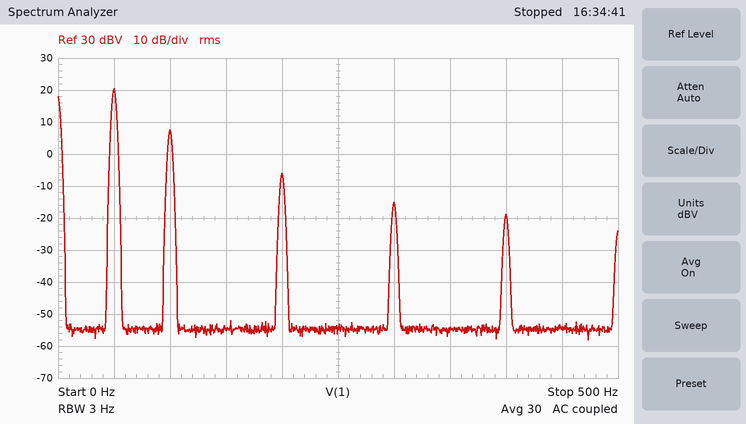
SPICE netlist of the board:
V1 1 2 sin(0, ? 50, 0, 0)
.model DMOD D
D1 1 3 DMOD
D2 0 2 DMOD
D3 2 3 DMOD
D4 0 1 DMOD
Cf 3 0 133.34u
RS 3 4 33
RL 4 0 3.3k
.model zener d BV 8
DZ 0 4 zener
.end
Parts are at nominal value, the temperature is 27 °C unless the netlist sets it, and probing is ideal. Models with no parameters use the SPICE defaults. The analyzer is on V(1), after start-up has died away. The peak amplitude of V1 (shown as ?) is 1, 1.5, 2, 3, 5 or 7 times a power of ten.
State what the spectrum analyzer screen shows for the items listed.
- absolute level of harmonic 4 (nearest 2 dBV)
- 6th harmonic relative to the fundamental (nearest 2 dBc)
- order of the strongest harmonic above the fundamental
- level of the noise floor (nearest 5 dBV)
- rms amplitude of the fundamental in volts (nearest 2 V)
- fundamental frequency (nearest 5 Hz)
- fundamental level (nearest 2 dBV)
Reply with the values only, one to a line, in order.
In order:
-6 dBV
-36 dBc
2
-55 dBV
10 V
50 Hz
20 dBV
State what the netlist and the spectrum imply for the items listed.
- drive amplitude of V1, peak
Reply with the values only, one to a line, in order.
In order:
30 V
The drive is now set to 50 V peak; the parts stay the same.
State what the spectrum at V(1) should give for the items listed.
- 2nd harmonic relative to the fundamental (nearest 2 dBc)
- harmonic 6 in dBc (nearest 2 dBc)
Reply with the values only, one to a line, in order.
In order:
-12 dBc
-34 dBc
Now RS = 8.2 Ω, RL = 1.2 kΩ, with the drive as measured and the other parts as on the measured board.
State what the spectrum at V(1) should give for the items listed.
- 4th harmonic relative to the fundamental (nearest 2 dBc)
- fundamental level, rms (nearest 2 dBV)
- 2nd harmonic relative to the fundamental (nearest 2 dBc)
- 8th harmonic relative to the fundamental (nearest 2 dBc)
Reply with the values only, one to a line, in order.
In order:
-34 dBc
20 dBV
-10 dBc
-38 dBc
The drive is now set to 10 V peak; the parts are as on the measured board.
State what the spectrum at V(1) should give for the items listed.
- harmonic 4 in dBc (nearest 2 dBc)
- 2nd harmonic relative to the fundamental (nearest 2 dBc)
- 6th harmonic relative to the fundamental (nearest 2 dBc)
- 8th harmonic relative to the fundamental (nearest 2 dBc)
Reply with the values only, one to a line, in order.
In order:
-42 dBc
-36 dBc
-46 dBc
-50 dBc
